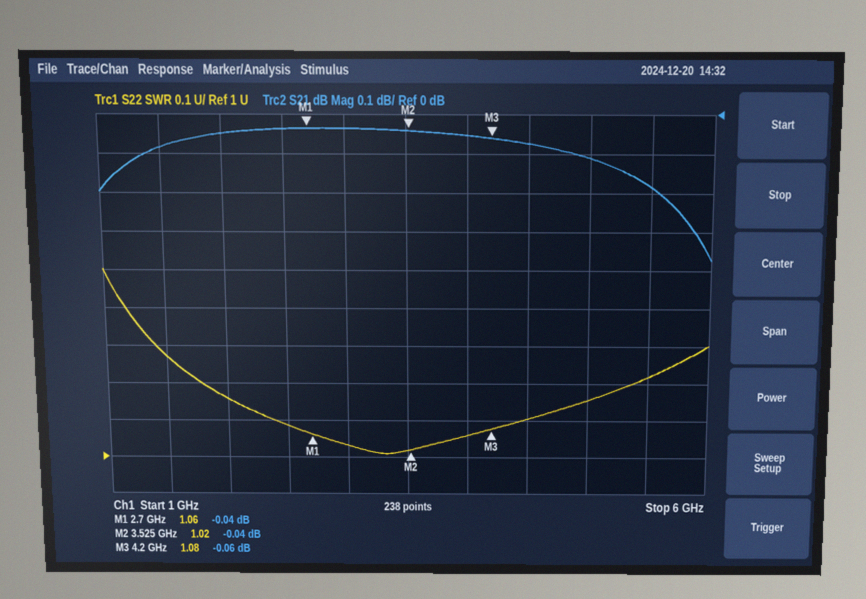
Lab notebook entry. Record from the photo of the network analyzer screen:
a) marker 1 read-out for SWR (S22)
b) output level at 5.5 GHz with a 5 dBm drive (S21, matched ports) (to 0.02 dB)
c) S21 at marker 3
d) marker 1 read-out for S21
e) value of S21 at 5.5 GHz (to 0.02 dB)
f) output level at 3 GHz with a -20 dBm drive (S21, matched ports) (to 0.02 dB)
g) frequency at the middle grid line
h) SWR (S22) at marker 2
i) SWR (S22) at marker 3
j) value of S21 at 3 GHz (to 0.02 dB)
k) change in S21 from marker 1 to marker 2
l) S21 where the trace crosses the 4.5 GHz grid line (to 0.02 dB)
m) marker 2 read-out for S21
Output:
1.06
4.82 dBm
-0.06 dB
-0.04 dB
-0.18 dB
-20.04 dBm
3.5 GHz
1.02
1.08
-0.04 dB
0.00 dB
-0.08 dB
-0.04 dB
